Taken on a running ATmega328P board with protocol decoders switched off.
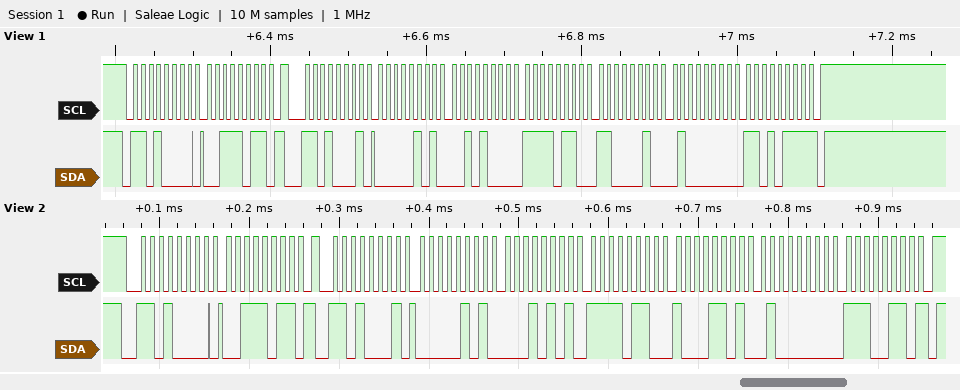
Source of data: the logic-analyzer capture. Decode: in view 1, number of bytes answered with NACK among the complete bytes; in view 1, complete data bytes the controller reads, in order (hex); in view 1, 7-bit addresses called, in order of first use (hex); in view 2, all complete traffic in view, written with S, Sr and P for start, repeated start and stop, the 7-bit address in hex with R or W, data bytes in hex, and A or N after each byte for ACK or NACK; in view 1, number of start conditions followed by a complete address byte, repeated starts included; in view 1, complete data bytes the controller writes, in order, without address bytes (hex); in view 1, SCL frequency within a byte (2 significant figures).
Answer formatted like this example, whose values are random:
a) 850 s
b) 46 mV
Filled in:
a) 1
b) 05 28 F6 C2 40 D7
c) 0x68
d) S 68W A 3B A Sr 68R A 05 A 15 A F6 A 8D A 40 A E6 N P
e) 2
f) 3B
g) 100 kHz
